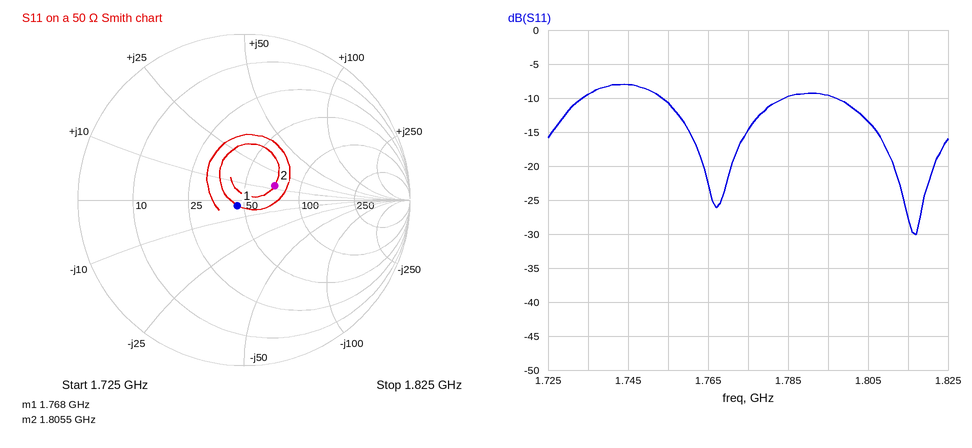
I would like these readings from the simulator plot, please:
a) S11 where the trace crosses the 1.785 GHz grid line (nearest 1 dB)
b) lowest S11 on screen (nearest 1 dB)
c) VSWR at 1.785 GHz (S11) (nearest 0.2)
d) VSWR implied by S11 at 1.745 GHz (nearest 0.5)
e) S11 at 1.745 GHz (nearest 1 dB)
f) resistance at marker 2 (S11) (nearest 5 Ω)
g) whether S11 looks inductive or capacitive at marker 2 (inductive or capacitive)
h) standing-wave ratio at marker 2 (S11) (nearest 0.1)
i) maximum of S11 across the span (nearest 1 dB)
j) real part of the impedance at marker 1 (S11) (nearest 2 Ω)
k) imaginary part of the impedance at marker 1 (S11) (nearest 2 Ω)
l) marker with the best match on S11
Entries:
-10 dB
-30 dB
2.0
2.5
-8 dB
70 Ω
inductive
1.5
-8 dB
46 Ω
-4 Ω
marker 1
